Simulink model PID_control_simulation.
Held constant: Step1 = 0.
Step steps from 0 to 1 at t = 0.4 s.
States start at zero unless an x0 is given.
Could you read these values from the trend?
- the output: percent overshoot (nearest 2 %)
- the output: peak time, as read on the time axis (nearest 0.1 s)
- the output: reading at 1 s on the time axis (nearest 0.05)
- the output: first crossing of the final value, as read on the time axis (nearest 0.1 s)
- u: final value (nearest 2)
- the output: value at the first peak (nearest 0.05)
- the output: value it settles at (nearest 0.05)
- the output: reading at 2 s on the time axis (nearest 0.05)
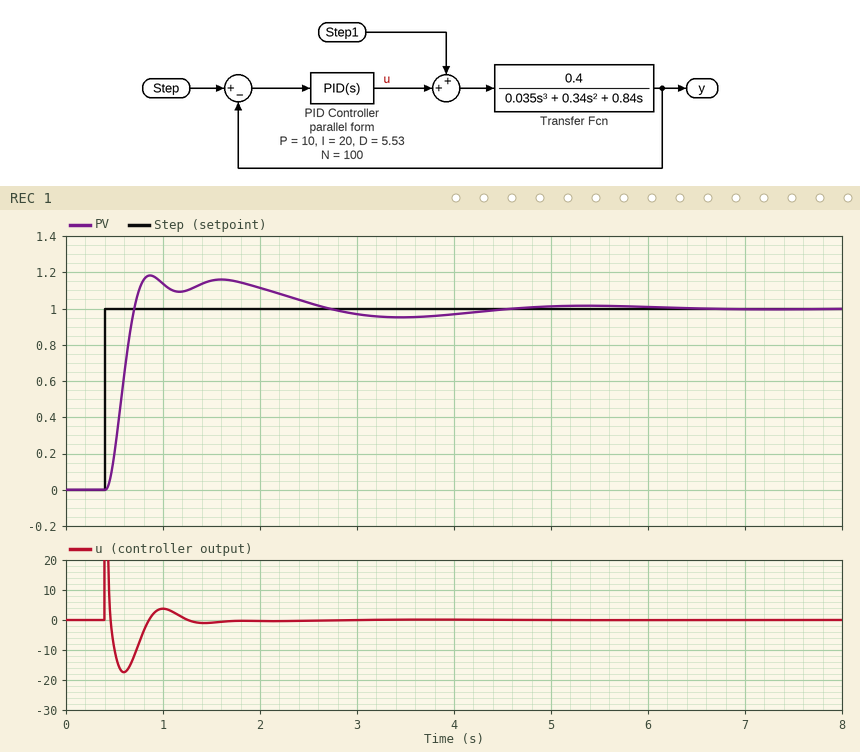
18 %
0.9 s
1.15
0.7 s
0
1.20
1.00
1.10
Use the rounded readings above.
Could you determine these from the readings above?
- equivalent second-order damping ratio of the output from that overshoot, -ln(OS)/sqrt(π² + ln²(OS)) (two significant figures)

0.48
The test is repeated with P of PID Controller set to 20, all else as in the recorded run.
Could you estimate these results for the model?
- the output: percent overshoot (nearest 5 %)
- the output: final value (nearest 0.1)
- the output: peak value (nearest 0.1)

35 %
1.0
1.4
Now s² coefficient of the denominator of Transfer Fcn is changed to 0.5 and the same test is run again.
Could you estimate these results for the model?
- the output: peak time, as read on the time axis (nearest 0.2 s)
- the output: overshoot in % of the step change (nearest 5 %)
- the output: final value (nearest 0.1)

1.4 s
25 %
1.0
